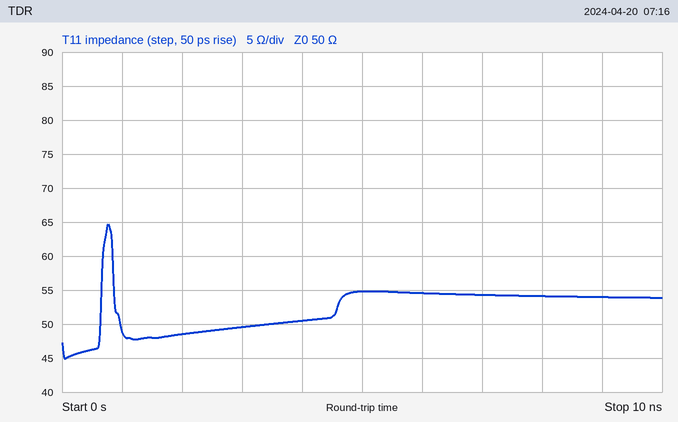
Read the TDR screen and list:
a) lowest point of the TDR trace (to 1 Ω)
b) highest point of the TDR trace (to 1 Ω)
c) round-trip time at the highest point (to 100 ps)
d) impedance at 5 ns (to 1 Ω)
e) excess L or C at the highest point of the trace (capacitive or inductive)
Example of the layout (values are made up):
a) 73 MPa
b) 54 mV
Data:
a) 45 Ω
b) 65 Ω
c) 800 ps
d) 55 Ω
e) inductive
